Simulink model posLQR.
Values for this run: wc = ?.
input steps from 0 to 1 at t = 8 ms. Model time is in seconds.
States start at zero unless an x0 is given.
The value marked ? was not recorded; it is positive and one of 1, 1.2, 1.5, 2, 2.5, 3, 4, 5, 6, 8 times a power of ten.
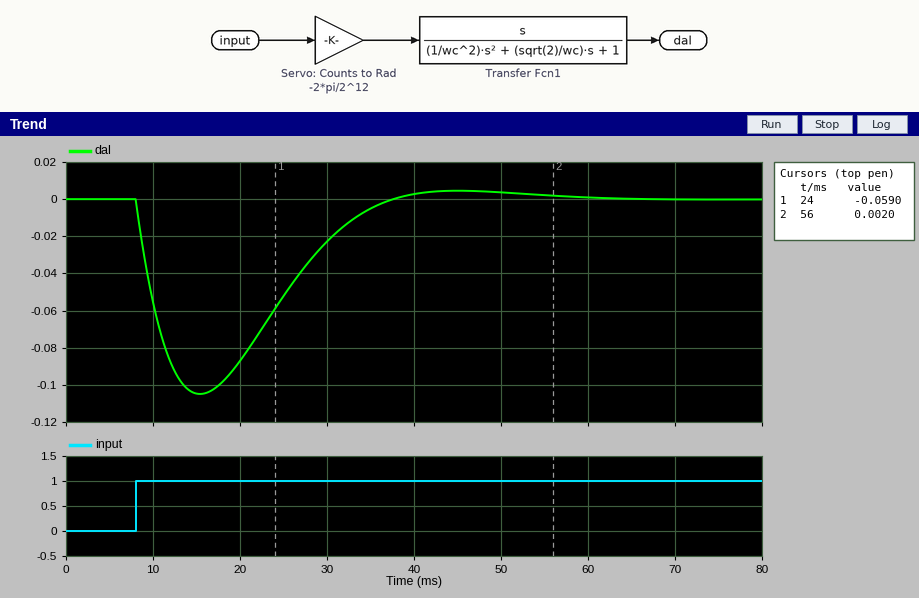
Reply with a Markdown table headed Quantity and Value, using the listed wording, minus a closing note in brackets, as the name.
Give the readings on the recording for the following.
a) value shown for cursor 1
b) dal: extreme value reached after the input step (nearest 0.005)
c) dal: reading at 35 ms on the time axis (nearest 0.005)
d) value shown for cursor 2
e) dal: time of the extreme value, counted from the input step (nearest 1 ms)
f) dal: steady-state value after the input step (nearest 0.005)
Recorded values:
| Quantity | Value |
|---|---|
| value shown for cursor 1 | -0.0590 |
| dal: extreme value reached after the input step | -0.105 |
| dal: reading at 35 ms on the time axis | -0.005 |
| value shown for cursor 2 | 0.0020 |
| dal: time of the extreme value, counted from the input step | 7 ms |
| dal: steady-state value after the input step | 0.000 |
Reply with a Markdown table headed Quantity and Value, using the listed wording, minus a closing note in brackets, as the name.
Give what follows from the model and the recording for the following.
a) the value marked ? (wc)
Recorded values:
| Quantity | Value |
|---|---|
| the value marked ? | 150 |
